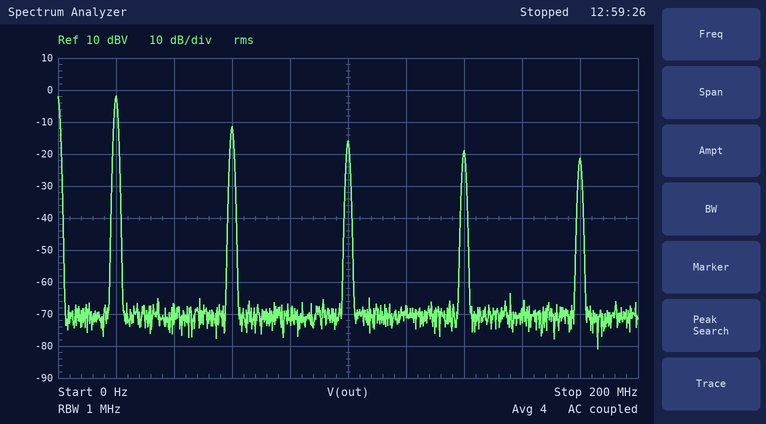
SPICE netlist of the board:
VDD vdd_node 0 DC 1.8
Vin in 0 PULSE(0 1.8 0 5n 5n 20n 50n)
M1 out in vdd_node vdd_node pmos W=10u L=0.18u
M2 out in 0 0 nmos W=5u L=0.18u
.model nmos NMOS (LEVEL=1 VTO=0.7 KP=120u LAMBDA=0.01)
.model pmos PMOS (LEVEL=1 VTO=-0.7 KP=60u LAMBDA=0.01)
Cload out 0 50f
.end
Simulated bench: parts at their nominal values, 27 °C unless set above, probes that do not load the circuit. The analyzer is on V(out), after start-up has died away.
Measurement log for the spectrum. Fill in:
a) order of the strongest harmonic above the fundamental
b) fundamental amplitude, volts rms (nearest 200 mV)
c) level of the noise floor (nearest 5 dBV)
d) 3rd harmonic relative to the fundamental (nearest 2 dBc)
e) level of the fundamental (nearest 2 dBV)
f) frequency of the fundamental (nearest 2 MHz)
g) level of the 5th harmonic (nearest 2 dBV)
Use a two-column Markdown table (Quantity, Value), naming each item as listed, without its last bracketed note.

| Quantity | Value |
|---|---|
| order of the strongest harmonic above the fundamental | 3 |
| fundamental amplitude, volts rms | 800 mV |
| level of the noise floor | -70 dBV |
| 3rd harmonic relative to the fundamental | -10 dBc |
| level of the fundamental | -2 dBV |
| frequency of the fundamental | 20 MHz |
| level of the 5th harmonic | -16 dBV |
